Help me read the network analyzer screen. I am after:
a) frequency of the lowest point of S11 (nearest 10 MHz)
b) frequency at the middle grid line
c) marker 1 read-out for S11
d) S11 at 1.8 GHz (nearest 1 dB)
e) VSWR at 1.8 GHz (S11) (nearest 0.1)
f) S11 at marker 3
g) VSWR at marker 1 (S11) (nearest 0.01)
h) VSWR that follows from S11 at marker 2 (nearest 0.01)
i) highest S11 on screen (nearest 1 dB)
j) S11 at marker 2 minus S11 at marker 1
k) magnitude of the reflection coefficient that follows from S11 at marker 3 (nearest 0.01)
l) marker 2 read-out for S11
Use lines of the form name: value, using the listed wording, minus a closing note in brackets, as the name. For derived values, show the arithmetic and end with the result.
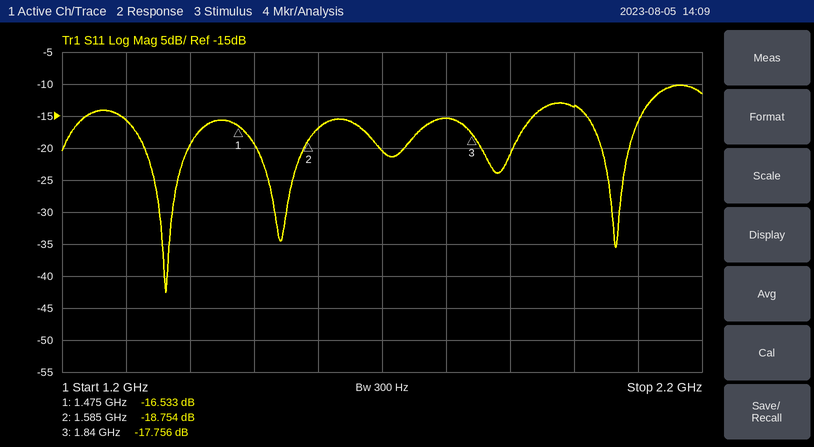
frequency of the lowest point of S11: 1.36 GHz
frequency at the middle grid line: 1.7 GHz
marker 1 read-out for S11: -16.533 dB
S11 at 1.8 GHz: -15 dB
VSWR at 1.8 GHz (S11): |Γ| = 10^(-15/20) = 0.1778; VSWR = (1 + 0.1778)/(1 − 0.1778) ≈ 1.4
S11 at marker 3: -17.756 dB
VSWR at marker 1 (S11): (1 + 0.1491)/(1 − 0.1491) ≈ 1.35
VSWR that follows from S11 at marker 2: (1 + 0.1154)/(1 − 0.1154) ≈ 1.26
highest S11 on screen: -10 dB
S11 at marker 2 minus S11 at marker 1: -18.754 − (-16.533) = -2.221 dB
magnitude of the reflection coefficient that follows from S11 at marker 3: 10^(-17.756/20) ≈ 0.13
marker 2 read-out for S11: -18.754 dB
